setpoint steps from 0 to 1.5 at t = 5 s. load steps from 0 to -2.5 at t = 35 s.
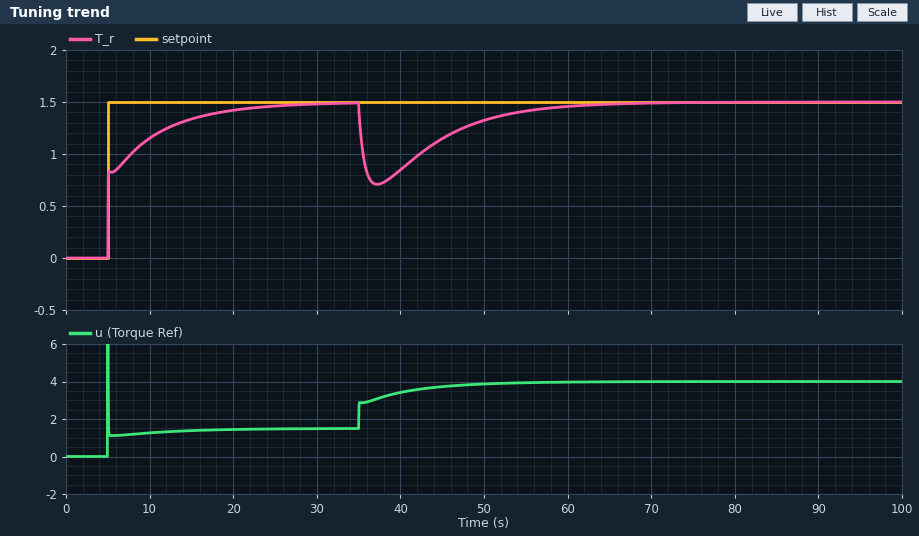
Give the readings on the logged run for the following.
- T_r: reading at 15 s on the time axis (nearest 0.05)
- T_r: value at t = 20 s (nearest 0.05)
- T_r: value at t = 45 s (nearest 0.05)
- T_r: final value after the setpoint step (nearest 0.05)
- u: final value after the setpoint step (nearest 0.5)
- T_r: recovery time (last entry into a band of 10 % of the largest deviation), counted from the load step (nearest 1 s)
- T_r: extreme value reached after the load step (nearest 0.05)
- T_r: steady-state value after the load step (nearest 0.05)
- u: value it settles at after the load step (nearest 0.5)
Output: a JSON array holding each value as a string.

["1.35", "1.40", "1.15", "1.50", "1.5", "21 s", "0.70", "1.50", "4.0"]
